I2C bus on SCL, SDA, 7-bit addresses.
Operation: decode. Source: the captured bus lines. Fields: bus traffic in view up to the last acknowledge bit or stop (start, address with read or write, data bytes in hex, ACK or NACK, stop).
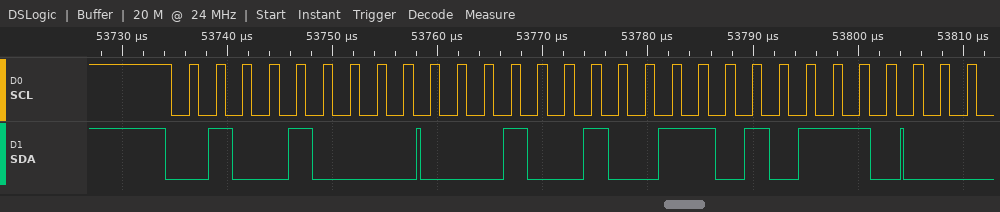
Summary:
start, address 24 write ACK, 12 ACK, D7 ACK
